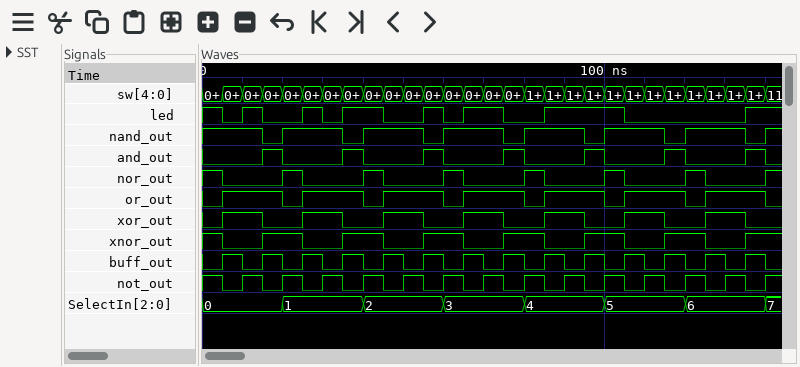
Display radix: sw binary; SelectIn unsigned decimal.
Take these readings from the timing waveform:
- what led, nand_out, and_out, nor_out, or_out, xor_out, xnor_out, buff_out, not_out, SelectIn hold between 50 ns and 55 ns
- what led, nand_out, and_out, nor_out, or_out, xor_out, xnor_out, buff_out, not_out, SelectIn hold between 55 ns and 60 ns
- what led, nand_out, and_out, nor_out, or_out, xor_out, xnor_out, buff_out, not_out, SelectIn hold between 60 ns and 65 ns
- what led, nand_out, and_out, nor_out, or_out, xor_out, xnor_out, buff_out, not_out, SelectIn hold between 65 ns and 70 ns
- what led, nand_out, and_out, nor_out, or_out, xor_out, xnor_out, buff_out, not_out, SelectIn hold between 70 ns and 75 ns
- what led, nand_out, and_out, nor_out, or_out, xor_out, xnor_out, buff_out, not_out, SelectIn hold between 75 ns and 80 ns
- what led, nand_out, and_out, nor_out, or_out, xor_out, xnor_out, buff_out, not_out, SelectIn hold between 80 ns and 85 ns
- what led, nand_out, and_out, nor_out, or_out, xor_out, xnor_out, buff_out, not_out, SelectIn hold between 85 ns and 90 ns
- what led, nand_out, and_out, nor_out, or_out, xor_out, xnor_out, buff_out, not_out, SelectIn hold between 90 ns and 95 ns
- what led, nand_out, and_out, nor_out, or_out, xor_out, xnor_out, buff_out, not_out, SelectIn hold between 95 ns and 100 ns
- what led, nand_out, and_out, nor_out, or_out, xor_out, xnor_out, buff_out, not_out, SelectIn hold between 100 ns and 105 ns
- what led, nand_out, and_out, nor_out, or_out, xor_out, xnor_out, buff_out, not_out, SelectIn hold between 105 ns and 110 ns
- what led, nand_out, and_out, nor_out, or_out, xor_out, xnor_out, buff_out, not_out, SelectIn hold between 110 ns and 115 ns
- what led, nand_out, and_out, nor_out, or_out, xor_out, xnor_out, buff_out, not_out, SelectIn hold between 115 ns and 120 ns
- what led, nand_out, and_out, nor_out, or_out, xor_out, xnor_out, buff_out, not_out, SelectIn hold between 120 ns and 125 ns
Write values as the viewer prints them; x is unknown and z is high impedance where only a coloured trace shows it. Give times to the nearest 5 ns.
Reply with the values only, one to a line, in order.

led=0, nand_out=1, and_out=0, nor_out=0, or_out=1, xor_out=1, xnor_out=0, buff_out=0, not_out=1, SelectIn=2
led=1, nand_out=0, and_out=1, nor_out=0, or_out=1, xor_out=0, xnor_out=1, buff_out=1, not_out=0, SelectIn=2
led=0, nand_out=1, and_out=0, nor_out=1, or_out=0, xor_out=0, xnor_out=1, buff_out=0, not_out=1, SelectIn=3
led=1, nand_out=1, and_out=0, nor_out=0, or_out=1, xor_out=1, xnor_out=0, buff_out=1, not_out=0, SelectIn=3
led=1, nand_out=1, and_out=0, nor_out=0, or_out=1, xor_out=1, xnor_out=0, buff_out=0, not_out=1, SelectIn=3
led=0, nand_out=0, and_out=1, nor_out=0, or_out=1, xor_out=0, xnor_out=1, buff_out=1, not_out=0, SelectIn=3
led=0, nand_out=1, and_out=0, nor_out=1, or_out=0, xor_out=0, xnor_out=1, buff_out=0, not_out=1, SelectIn=4
led=1, nand_out=1, and_out=0, nor_out=0, or_out=1, xor_out=1, xnor_out=0, buff_out=1, not_out=0, SelectIn=4
led=1, nand_out=1, and_out=0, nor_out=0, or_out=1, xor_out=1, xnor_out=0, buff_out=0, not_out=1, SelectIn=4
led=1, nand_out=0, and_out=1, nor_out=0, or_out=1, xor_out=0, xnor_out=1, buff_out=1, not_out=0, SelectIn=4
led=1, nand_out=1, and_out=0, nor_out=1, or_out=0, xor_out=0, xnor_out=1, buff_out=0, not_out=1, SelectIn=5
led=0, nand_out=1, and_out=0, nor_out=0, or_out=1, xor_out=1, xnor_out=0, buff_out=1, not_out=0, SelectIn=5
led=0, nand_out=1, and_out=0, nor_out=0, or_out=1, xor_out=1, xnor_out=0, buff_out=0, not_out=1, SelectIn=5
led=0, nand_out=0, and_out=1, nor_out=0, or_out=1, xor_out=0, xnor_out=1, buff_out=1, not_out=0, SelectIn=5
led=0, nand_out=1, and_out=0, nor_out=1, or_out=0, xor_out=0, xnor_out=1, buff_out=0, not_out=1, SelectIn=6
